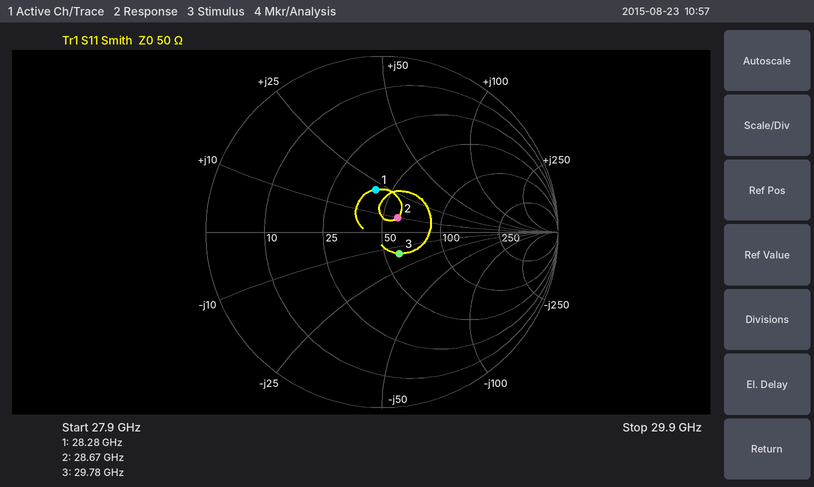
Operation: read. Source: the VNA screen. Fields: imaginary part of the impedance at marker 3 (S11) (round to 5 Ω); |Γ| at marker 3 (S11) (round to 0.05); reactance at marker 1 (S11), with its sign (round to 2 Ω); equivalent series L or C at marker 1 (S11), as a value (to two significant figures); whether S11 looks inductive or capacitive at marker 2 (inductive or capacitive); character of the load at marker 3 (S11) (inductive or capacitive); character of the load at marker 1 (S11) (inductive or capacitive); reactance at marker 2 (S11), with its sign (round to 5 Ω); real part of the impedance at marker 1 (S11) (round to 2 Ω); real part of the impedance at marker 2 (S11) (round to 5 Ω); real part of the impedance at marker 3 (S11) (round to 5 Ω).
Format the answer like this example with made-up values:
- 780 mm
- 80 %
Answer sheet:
- -15 Ω
- 0.15
- +22 Ω
- 120 pH
- inductive
- capacitive
- inductive
- +10 Ω
- 42 Ω
- 60 Ω
- 60 Ω
